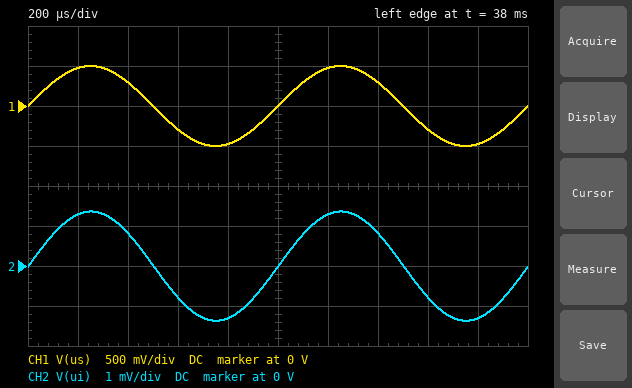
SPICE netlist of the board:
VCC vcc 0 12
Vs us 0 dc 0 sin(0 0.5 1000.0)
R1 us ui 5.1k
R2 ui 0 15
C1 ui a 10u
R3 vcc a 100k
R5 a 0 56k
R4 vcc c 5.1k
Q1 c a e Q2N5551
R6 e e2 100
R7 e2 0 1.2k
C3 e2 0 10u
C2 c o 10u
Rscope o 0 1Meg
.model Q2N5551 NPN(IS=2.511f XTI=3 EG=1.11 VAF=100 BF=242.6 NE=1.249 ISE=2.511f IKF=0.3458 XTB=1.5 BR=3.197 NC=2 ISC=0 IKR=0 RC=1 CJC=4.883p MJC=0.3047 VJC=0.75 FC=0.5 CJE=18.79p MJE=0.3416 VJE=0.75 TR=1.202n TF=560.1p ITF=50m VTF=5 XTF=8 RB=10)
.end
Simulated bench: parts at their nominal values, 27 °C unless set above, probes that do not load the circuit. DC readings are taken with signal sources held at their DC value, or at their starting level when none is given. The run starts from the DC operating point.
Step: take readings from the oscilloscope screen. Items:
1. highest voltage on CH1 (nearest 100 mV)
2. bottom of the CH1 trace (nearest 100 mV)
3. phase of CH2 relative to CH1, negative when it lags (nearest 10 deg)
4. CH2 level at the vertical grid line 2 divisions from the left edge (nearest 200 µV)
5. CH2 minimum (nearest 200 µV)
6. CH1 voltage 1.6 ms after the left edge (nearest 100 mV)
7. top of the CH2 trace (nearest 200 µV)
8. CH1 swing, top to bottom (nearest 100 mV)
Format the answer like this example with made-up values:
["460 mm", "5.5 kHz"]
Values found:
["500 mV", "-500 mV", "0 deg", "800 µV", "-1.4 mV", "-300 mV", "1.4 mV", "1.0 V"]
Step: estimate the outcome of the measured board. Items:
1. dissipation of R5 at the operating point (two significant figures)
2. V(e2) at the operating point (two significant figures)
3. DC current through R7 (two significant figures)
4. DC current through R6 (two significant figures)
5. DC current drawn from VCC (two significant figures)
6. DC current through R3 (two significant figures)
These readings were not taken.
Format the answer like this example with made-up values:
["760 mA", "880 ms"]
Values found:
["180 µW", "2.3 V", "1.9 mA", "1.9 mA", "1.9 mA", "88 µA"]
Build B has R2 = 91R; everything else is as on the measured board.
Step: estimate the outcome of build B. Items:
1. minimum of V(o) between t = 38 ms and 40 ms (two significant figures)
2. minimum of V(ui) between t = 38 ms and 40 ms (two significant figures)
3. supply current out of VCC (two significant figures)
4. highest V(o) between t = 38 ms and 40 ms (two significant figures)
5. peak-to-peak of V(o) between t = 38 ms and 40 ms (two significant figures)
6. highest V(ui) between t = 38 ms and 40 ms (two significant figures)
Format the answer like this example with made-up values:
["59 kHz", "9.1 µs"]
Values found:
["-30 mV", "-7.2 mV", "1.9 mA", "230 mV", "260 mV", "6.2 mV"]
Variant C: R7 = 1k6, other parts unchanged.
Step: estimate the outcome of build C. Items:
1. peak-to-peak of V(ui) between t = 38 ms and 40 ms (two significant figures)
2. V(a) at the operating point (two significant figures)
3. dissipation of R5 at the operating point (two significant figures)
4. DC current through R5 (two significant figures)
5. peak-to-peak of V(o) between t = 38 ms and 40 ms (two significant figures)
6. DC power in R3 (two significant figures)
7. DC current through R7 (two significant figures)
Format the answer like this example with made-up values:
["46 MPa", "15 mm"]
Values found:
["2.8 mV", "3.7 V", "240 µW", "66 µA", "78 mV", "690 µW", "1.8 mA"]
